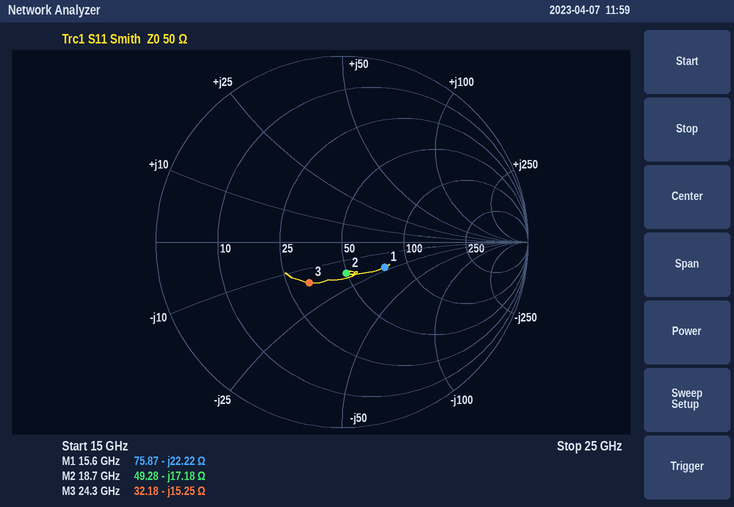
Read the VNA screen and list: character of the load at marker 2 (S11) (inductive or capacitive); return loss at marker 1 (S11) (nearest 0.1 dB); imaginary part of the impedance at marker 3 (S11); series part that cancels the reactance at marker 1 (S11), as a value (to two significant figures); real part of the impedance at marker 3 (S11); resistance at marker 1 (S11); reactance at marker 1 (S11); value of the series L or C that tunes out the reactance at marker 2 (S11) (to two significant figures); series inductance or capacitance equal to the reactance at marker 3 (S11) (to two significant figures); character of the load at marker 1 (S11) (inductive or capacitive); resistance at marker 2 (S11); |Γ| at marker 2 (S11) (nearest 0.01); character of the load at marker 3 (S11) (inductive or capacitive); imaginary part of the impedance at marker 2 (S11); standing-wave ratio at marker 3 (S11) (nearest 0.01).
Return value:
capacitive
11.5 dB
-15.25 Ω
230 pH
32.18 Ω
75.87 Ω
-22.22 Ω
150 pH
430 fF
capacitive
49.28 Ω
0.17
capacitive
-17.18 Ω
1.78
